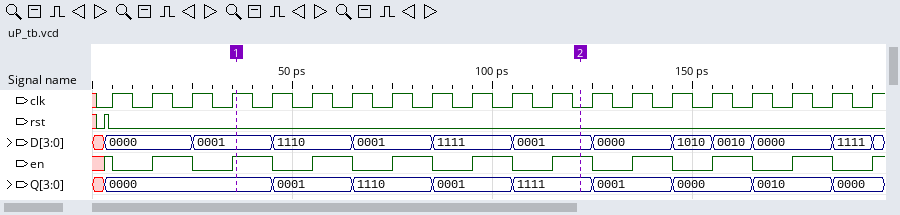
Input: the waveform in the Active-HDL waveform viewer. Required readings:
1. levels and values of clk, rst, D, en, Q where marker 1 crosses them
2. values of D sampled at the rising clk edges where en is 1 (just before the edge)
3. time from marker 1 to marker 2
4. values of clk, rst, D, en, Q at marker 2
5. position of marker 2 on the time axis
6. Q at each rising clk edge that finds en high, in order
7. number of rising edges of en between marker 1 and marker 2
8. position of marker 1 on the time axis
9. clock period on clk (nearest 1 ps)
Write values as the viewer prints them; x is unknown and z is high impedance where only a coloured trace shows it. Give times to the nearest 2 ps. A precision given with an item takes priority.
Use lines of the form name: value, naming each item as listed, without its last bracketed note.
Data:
levels and values of clk, rst, D, en, Q where marker 1 crosses them: clk=1, rst=0, D=0001, en=1, Q=0000
values of D sampled at the rising clk edges where en is 1: 0000, 0000, 0001, 1110, 0001, 1111, 0001, 0000, 0010, 0000
time from marker 1 to marker 2: 86 ps
values of clk, rst, D, en, Q at marker 2: clk=0, rst=0, D=0001, en=1, Q=1111
position of marker 2 on the time axis: 122 ps
Q at each rising clk edge that finds en high, in order: 0000, 0000, 0000, 0001, 1110, 0001, 1111, 0001, 0000, 0010
number of rising edges of en between marker 1 and marker 2: 4
position of marker 1 on the time axis: 36 ps
clock period on clk: 10 ps
